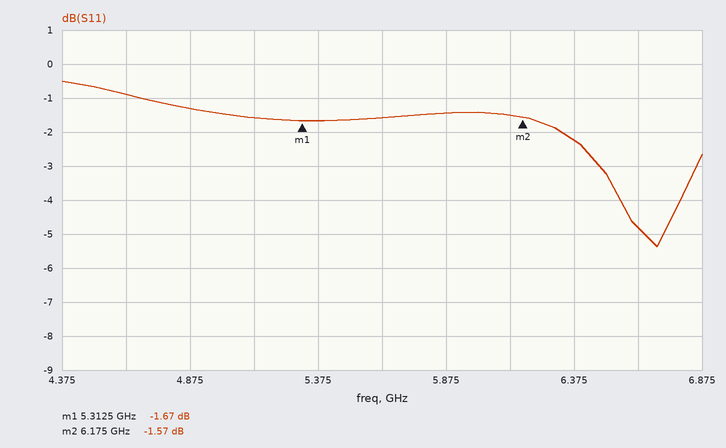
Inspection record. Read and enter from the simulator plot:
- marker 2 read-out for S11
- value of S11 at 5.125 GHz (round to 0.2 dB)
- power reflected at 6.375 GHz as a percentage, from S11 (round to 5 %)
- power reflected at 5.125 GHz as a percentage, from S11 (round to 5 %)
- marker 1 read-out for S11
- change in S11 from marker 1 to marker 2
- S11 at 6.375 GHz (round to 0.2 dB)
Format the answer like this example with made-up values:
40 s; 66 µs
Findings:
-1.57 dB; -1.6 dB; 60 %; 70 %; -1.67 dB; 0.10 dB; -2.2 dB
